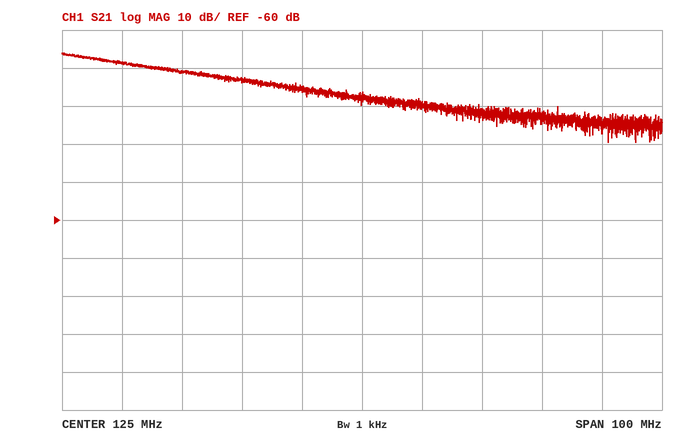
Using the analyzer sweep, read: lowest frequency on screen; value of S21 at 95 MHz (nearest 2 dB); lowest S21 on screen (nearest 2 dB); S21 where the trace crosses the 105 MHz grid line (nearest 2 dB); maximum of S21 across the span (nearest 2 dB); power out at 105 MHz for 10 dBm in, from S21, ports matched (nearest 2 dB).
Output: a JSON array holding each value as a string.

["75 MHz", "-20 dB", "-40 dB", "-24 dB", "-16 dB", "-14 dBm"]
